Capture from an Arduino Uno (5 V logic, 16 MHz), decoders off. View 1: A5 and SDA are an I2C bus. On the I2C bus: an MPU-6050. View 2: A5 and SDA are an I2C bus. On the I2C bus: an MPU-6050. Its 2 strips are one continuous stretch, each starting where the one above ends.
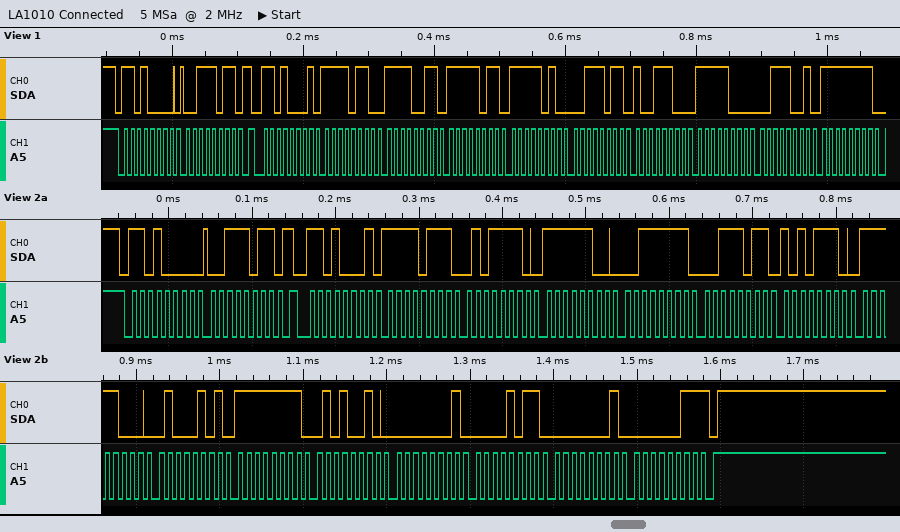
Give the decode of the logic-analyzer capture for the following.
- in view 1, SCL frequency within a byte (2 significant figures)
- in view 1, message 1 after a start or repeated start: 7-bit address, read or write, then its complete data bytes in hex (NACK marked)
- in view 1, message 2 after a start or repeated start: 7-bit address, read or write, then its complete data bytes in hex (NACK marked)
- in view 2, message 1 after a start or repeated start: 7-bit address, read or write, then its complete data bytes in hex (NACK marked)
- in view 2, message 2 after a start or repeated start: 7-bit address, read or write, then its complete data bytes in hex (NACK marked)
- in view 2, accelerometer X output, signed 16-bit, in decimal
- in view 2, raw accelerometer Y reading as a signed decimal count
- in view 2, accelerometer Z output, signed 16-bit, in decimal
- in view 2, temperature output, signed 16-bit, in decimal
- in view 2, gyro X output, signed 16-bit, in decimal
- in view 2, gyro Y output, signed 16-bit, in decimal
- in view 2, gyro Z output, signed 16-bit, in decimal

100 kHz
0x68 write: 3B
0x68 read: F6 F3 FB FA 3B 9C F8 39 FF
0x68 write: 3B
0x68 read: F7 5E FC 3F 3B AE F8 45 FF 52 01 0B 01 03 NACK
-2210
-961
15278
-1979
-174
267
259
